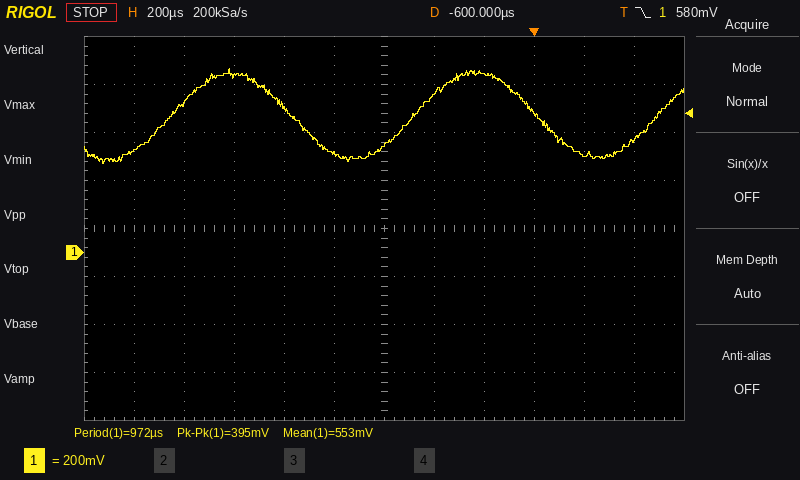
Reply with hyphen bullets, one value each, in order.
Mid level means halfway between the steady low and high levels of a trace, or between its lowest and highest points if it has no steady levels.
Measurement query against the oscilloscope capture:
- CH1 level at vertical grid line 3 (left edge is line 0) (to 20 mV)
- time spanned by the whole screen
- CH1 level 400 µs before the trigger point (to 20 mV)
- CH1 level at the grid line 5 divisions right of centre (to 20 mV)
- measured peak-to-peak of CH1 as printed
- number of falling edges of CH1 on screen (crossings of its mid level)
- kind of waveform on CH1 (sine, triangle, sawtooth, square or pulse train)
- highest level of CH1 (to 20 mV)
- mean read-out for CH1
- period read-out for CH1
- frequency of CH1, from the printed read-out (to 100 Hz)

- 740 mV
- 2.4 ms
- 660 mV
- 480 mV
- 395 mV
- 2
- sine
- 760 mV
- 553 mV
- 972 µs
- 1.0 kHz
